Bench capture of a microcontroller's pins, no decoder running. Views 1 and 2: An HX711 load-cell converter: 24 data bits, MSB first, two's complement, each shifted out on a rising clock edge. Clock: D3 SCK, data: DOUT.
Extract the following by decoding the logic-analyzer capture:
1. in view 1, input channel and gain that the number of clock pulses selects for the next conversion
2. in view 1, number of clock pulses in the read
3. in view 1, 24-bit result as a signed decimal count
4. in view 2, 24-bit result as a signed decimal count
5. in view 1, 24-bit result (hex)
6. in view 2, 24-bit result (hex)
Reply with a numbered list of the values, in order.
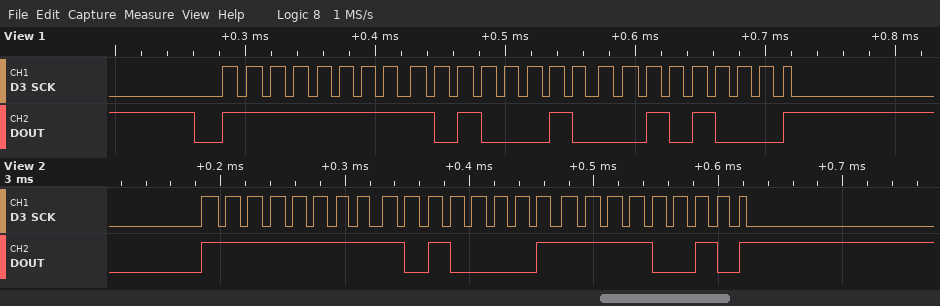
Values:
1. channel A, gain 128
2. 25
3. -24024
4. -24078
5. 0xFFA228
6. 0xFFA1F2
